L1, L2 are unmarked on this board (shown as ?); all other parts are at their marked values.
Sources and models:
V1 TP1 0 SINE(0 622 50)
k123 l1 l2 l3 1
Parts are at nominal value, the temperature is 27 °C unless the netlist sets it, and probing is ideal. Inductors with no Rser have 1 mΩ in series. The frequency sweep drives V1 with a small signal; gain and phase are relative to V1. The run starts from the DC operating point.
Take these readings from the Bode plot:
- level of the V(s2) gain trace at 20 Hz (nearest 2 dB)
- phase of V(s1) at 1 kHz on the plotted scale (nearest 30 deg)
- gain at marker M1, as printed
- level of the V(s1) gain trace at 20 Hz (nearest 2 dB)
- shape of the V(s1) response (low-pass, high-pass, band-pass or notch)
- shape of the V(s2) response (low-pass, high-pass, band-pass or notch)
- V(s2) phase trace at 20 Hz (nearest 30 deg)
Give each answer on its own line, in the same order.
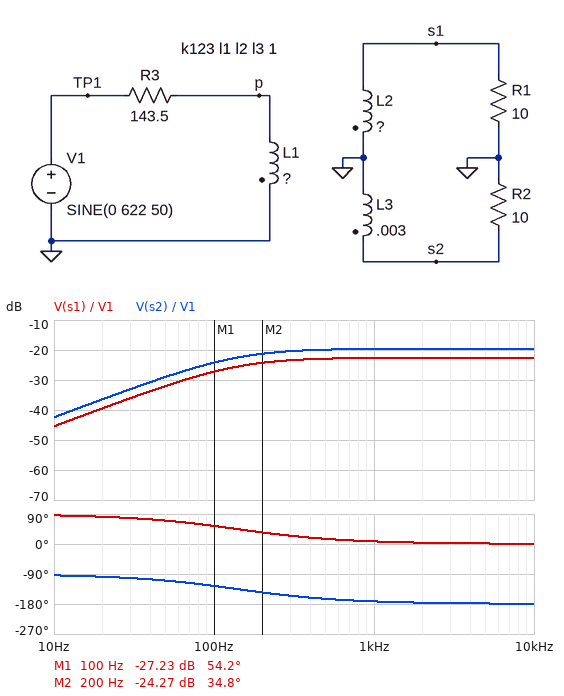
-36 dB
0 deg
-27.23 dB
-40 dB
high-pass
high-pass
-90 deg
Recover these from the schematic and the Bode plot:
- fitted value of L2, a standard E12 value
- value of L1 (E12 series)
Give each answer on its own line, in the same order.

1.5 mH
100 mH
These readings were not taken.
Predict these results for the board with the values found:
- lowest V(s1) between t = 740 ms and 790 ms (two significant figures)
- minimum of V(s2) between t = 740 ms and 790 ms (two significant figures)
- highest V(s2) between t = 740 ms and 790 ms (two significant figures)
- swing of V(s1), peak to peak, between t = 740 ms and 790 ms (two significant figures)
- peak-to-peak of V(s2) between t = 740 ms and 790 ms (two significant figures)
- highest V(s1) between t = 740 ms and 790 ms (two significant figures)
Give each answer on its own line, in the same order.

-16 V
-22 V
22 V
31 V
44 V
16 V
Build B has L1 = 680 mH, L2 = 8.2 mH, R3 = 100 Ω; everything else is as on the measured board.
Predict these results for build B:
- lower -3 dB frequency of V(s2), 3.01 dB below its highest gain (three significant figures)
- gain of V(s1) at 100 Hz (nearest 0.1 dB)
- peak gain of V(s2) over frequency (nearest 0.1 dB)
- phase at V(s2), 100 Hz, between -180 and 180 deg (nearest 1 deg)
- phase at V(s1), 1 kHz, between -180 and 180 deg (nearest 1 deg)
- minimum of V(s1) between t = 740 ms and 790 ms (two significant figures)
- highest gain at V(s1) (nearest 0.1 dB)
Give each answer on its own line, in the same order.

20.1 Hz
-20.7 dB
-24.9 dB
-169 deg
1 deg
-54 V
-20.5 dB
